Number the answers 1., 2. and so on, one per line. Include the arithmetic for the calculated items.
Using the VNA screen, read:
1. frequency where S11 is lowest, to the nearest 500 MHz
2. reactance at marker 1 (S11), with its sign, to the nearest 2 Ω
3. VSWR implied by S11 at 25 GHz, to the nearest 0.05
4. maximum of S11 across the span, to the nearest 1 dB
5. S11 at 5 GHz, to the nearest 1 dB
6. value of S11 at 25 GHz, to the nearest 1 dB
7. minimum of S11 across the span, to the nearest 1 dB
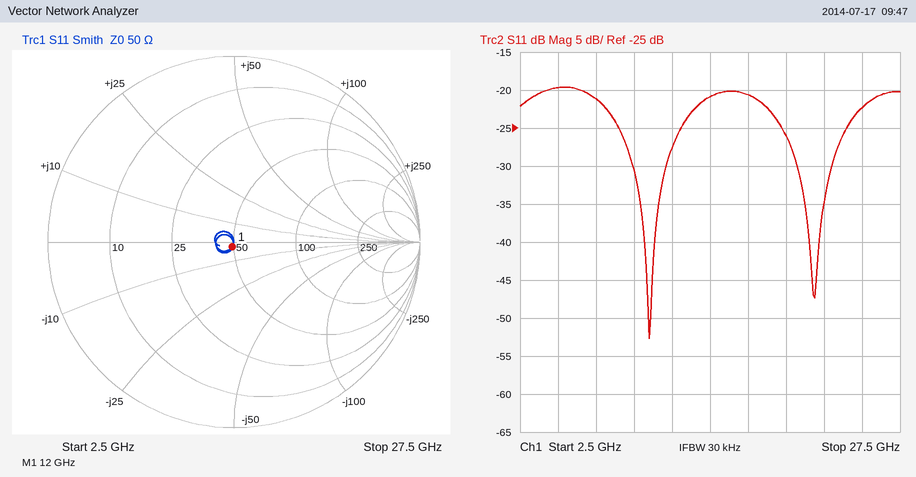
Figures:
1. 11.0 GHz
2. -2 Ω
3. |Γ| = 10^(-22/20) = 0.0794; VSWR = (1 + 0.0794)/(1 − 0.0794) ≈ 1.17, so 1.15 to the nearest 0.05
4. -20 dB
5. -20 dB
6. -22 dB
7. -53 dB
